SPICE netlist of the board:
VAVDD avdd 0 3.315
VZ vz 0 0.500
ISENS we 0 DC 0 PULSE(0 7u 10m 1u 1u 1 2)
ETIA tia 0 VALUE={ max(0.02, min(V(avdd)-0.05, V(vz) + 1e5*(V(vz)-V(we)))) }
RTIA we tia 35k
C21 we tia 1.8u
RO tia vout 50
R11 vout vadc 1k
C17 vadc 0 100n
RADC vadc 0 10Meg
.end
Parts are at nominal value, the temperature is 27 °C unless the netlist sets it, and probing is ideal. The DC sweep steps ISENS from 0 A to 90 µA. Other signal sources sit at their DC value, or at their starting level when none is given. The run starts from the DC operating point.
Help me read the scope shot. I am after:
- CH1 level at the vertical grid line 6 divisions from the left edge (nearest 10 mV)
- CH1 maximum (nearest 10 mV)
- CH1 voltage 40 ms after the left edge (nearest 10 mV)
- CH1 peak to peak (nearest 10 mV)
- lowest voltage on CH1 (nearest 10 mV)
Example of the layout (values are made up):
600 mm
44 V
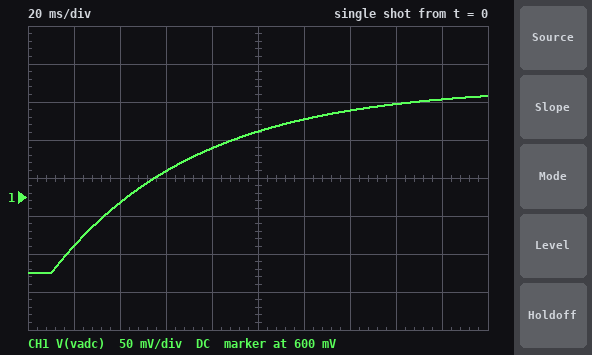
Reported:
700 mV
730 mV
590 mV
230 mV
500 mV
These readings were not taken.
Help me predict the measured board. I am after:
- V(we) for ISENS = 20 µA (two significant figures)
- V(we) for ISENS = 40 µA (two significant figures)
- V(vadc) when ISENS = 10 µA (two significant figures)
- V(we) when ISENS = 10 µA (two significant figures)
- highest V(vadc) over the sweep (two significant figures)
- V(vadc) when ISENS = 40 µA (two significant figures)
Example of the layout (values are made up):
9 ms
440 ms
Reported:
500 mV
500 mV
850 mV
500 mV
3.3 V
1.9 V
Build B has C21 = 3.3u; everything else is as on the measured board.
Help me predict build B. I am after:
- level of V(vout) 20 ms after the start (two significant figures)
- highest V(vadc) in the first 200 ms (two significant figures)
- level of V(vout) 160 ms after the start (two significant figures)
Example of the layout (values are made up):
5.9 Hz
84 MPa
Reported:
520 mV
700 mV
680 mV
